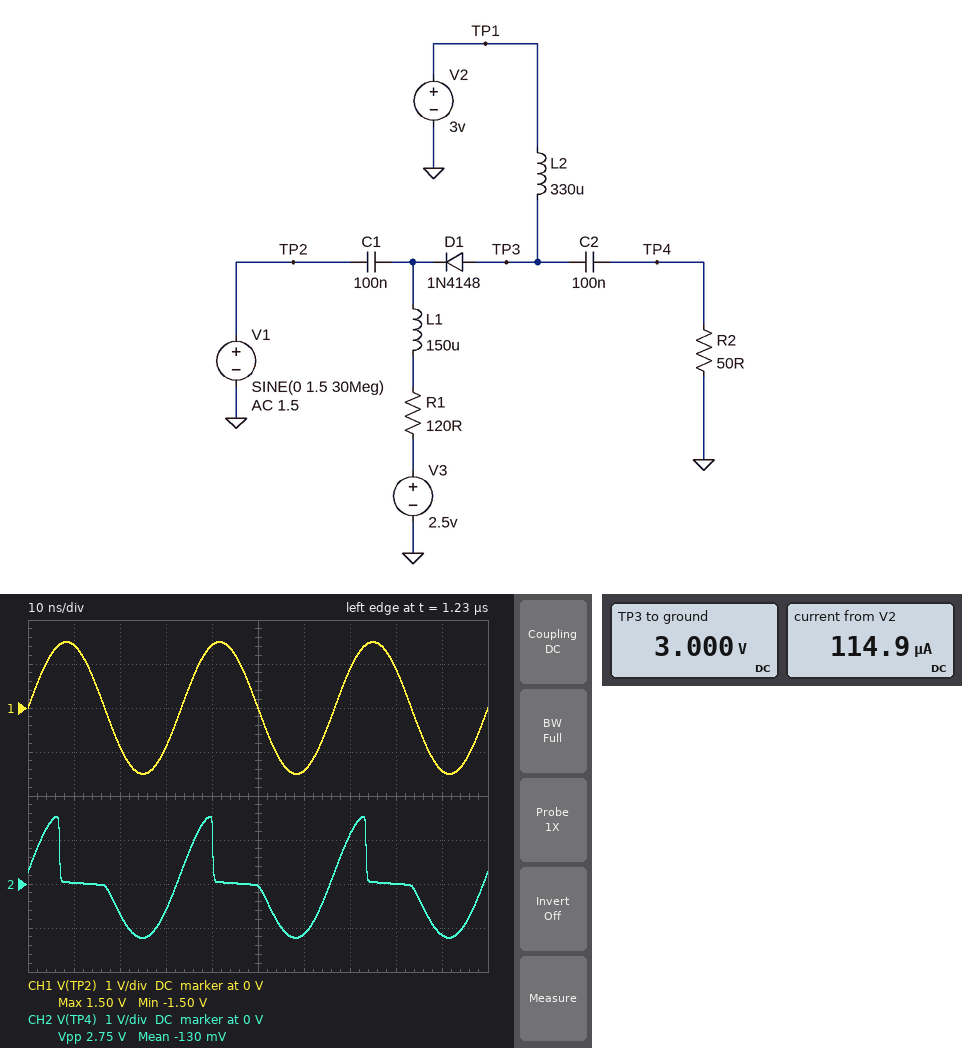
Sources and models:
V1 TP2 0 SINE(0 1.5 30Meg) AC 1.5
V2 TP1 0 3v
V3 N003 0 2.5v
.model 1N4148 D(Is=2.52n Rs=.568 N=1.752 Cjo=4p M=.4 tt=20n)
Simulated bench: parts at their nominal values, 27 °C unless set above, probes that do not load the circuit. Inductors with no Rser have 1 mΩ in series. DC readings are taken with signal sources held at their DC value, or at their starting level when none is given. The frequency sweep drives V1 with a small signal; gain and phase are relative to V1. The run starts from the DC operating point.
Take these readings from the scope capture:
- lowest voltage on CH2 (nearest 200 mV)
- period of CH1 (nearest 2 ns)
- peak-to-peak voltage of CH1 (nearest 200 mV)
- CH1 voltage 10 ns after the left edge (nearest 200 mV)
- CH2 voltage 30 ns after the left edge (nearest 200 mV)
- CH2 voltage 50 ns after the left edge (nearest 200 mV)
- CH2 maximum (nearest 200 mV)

-1.2 V
34 ns
3.0 V
1.4 V
-600 mV
0 V
1.6 V
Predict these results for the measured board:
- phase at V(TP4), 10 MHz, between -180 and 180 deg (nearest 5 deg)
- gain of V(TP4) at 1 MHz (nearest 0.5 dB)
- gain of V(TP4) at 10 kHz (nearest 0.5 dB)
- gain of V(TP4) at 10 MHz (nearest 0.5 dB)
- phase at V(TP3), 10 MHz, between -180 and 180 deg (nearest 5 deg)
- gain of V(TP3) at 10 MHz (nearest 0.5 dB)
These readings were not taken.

45 deg
-19.0 dB
-40.5 dB
-14.5 dB
45 deg
-14.5 dB
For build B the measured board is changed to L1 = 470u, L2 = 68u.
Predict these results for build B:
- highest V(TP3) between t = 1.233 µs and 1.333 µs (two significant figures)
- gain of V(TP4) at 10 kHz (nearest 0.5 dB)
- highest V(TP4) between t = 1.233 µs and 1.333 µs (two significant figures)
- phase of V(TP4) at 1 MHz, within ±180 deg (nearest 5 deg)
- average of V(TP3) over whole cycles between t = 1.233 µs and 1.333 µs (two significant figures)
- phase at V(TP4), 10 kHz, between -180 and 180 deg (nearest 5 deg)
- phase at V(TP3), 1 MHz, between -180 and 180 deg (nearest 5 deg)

4.6 V
-54.5 dB
1.6 V
15 deg
2.9 V
-130 deg
10 deg
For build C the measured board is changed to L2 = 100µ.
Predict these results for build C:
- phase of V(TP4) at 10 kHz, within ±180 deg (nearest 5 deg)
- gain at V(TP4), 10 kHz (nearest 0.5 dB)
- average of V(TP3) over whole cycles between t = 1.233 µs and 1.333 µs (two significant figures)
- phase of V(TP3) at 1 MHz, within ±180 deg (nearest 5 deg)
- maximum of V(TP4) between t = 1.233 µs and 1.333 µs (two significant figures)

-135 deg
-52.0 dB
2.9 V
10 deg
1.6 V
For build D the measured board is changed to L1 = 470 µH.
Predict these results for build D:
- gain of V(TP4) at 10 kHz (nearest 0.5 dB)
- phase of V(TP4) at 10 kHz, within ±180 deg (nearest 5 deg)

-40.0 dB
-135 deg
